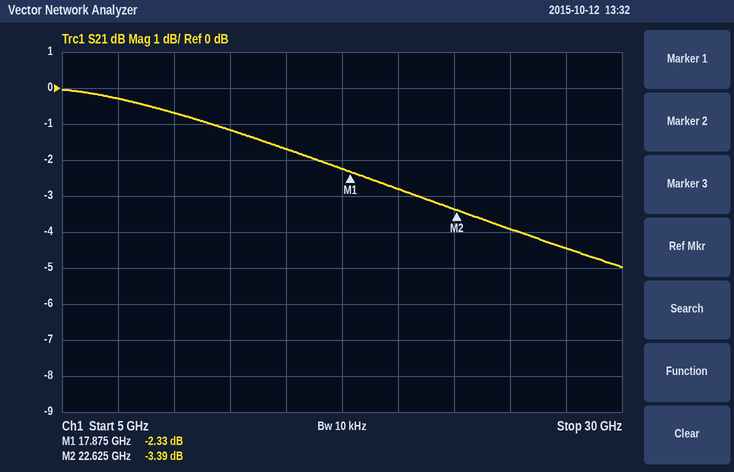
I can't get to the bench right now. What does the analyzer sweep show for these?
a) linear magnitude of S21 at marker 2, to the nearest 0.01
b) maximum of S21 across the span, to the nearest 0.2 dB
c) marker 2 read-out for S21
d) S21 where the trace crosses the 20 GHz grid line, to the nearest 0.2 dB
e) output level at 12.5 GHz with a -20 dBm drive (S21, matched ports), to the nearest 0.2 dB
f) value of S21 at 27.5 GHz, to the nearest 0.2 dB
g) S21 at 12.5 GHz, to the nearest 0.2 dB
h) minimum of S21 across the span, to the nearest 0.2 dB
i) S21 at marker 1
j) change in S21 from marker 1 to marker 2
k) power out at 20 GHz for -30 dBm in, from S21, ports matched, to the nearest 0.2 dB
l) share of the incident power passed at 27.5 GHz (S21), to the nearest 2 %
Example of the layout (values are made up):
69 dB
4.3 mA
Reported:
0.68
0.0 dB
-3.39 dB
-2.8 dB
-21.2 dBm
-4.4 dB
-1.2 dB
-5.0 dB
-2.33 dB
-1.06 dB
-32.8 dBm
36 %
